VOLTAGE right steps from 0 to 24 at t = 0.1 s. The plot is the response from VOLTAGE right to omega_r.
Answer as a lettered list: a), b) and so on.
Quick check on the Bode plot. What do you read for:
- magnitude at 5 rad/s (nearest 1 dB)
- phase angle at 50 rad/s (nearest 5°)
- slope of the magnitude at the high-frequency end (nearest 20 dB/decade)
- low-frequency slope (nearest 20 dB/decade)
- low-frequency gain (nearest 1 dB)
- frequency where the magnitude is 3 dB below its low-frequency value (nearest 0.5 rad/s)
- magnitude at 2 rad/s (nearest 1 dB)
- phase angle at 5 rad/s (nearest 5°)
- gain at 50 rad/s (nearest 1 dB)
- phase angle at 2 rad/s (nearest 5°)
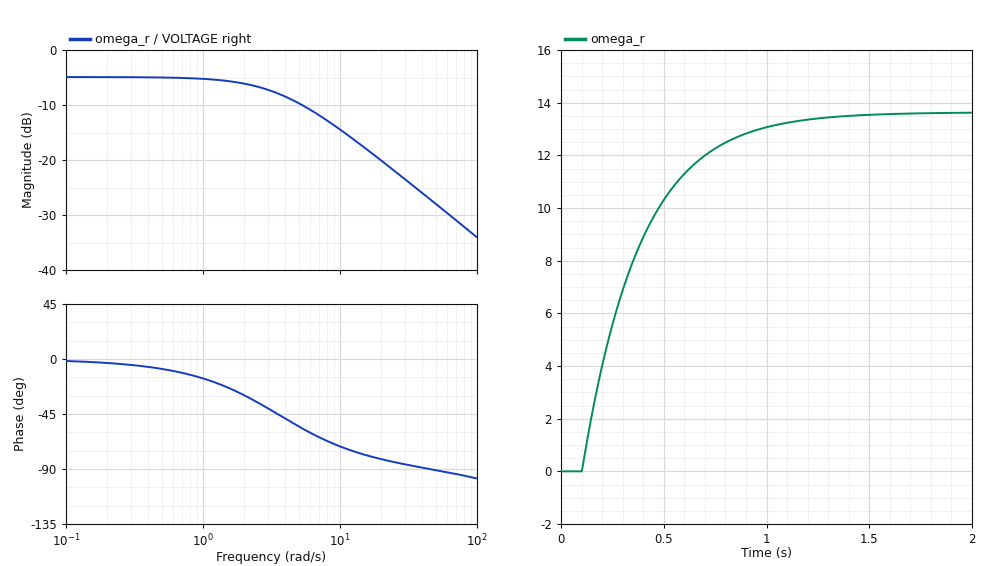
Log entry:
a) -10 dB
b) -90°
c) -20 dB/decade
d) 0 dB/decade
e) -5 dB
f) 3.5 rad/s
g) -6 dB
h) -55°
i) -28 dB
j) -30°
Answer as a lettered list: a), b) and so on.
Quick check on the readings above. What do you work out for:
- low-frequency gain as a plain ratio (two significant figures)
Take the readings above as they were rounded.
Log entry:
a) 0.56
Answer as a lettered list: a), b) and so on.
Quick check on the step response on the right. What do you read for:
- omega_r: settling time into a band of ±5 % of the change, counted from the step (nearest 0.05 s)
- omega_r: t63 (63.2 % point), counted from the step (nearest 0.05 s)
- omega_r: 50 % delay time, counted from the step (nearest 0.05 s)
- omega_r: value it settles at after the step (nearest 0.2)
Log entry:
a) 0.85 s
b) 0.30 s
c) 0.20 s
d) 13.6
